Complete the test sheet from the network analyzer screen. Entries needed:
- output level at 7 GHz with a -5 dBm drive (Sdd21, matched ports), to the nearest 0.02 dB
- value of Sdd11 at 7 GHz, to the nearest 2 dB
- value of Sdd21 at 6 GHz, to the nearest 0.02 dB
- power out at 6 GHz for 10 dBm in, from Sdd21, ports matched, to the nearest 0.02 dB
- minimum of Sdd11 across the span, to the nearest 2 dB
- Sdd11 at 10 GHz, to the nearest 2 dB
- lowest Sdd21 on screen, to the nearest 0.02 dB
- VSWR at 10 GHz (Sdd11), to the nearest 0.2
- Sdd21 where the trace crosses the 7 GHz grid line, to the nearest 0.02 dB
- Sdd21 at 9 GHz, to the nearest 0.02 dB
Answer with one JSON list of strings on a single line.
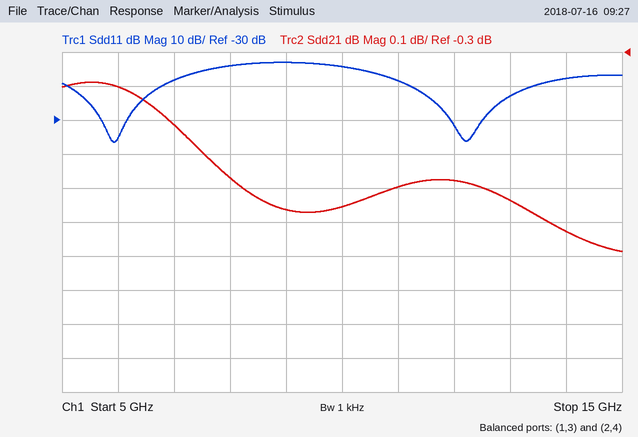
["-5.52 dBm", "-18 dB", "-0.40 dB", "9.60 dBm", "-36 dB", "-14 dB", "-0.88 dB", "1.4", "-0.52 dB", "-0.76 dB"]
